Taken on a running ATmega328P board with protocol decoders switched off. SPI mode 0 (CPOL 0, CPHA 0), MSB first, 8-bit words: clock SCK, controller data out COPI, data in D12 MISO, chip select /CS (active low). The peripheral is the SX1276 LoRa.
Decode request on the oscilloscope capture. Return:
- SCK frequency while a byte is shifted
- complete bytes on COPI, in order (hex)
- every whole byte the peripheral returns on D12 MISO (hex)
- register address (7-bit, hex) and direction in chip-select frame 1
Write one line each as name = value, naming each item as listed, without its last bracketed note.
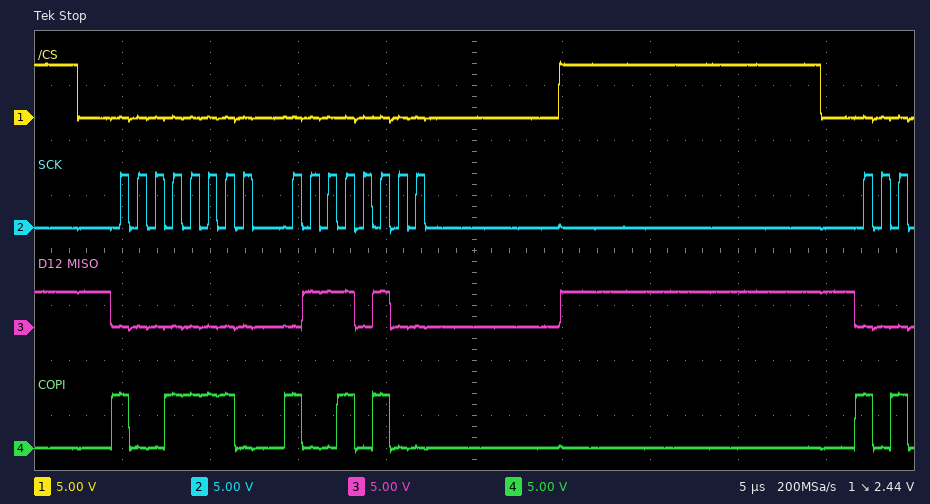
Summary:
SCK frequency while a byte is shifted = 1 MHz
complete bytes on COPI, in order = 9E 94
every whole byte the peripheral returns on D12 MISO = 00 74
register address (7-bit, hex) and direction in chip-select frame 1 = 0x1E write
